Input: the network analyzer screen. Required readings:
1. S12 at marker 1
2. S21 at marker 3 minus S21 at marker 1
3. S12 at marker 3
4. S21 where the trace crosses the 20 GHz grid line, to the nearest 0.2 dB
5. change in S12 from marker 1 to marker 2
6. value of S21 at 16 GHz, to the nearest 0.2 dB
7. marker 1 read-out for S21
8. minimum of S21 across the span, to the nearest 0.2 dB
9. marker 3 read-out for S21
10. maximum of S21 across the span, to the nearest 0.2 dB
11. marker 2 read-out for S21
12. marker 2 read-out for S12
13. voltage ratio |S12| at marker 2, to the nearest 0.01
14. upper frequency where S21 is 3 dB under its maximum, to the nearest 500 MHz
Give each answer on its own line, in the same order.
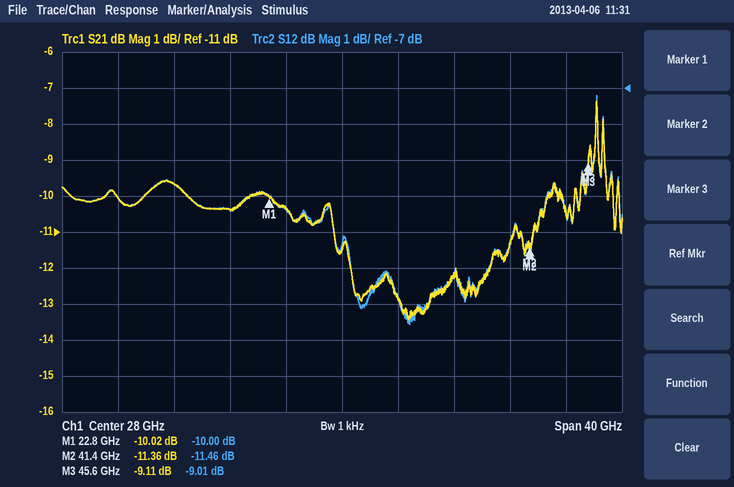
-10.00 dB
0.91 dB
-9.01 dB
-10.4 dB
-1.46 dB
-9.6 dB
-10.02 dB
-13.4 dB
-9.11 dB
-7.4 dB
-11.36 dB
-11.46 dB
0.27
47.5 GHz
